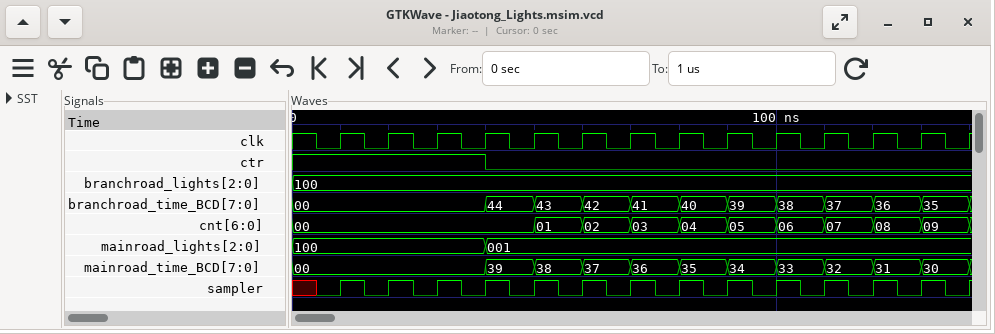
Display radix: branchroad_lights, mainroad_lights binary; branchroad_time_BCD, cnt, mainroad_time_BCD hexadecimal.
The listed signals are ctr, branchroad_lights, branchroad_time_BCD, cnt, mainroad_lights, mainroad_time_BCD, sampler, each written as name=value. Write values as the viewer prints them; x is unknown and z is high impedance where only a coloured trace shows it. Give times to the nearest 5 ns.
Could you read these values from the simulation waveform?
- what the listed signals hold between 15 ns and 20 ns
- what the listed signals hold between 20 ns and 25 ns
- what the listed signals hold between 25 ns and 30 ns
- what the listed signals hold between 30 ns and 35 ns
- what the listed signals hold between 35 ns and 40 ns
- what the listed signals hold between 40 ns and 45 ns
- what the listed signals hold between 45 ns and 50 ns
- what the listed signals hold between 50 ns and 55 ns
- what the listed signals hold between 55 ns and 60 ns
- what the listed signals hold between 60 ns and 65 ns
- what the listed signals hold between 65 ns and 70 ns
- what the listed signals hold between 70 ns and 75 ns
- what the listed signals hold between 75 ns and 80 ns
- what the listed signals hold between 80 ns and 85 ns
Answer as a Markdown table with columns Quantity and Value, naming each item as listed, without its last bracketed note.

| Quantity | Value |
|---|---|
| what the listed signals hold between 15 ns and 20 ns | ctr=1, branchroad_lights=100, branchroad_time_BCD=00, cnt=00, mainroad_lights=100, mainroad_time_BCD=00, sampler=0 |
| what the listed signals hold between 20 ns and 25 ns | ctr=1, branchroad_lights=100, branchroad_time_BCD=00, cnt=00, mainroad_lights=100, mainroad_time_BCD=00, sampler=1 |
| what the listed signals hold between 25 ns and 30 ns | ctr=1, branchroad_lights=100, branchroad_time_BCD=00, cnt=00, mainroad_lights=100, mainroad_time_BCD=00, sampler=0 |
| what the listed signals hold between 30 ns and 35 ns | ctr=1, branchroad_lights=100, branchroad_time_BCD=00, cnt=00, mainroad_lights=100, mainroad_time_BCD=00, sampler=1 |
| what the listed signals hold between 35 ns and 40 ns | ctr=1, branchroad_lights=100, branchroad_time_BCD=00, cnt=00, mainroad_lights=100, mainroad_time_BCD=00, sampler=0 |
| what the listed signals hold between 40 ns and 45 ns | ctr=0, branchroad_lights=100, branchroad_time_BCD=44, cnt=00, mainroad_lights=001, mainroad_time_BCD=39, sampler=1 |
| what the listed signals hold between 45 ns and 50 ns | ctr=0, branchroad_lights=100, branchroad_time_BCD=44, cnt=00, mainroad_lights=001, mainroad_time_BCD=39, sampler=0 |
| what the listed signals hold between 50 ns and 55 ns | ctr=0, branchroad_lights=100, branchroad_time_BCD=43, cnt=01, mainroad_lights=001, mainroad_time_BCD=38, sampler=1 |
| what the listed signals hold between 55 ns and 60 ns | ctr=0, branchroad_lights=100, branchroad_time_BCD=43, cnt=01, mainroad_lights=001, mainroad_time_BCD=38, sampler=0 |
| what the listed signals hold between 60 ns and 65 ns | ctr=0, branchroad_lights=100, branchroad_time_BCD=42, cnt=02, mainroad_lights=001, mainroad_time_BCD=37, sampler=1 |
| what the listed signals hold between 65 ns and 70 ns | ctr=0, branchroad_lights=100, branchroad_time_BCD=42, cnt=02, mainroad_lights=001, mainroad_time_BCD=37, sampler=0 |
| what the listed signals hold between 70 ns and 75 ns | ctr=0, branchroad_lights=100, branchroad_time_BCD=41, cnt=03, mainroad_lights=001, mainroad_time_BCD=36, sampler=1 |
| what the listed signals hold between 75 ns and 80 ns | ctr=0, branchroad_lights=100, branchroad_time_BCD=41, cnt=03, mainroad_lights=001, mainroad_time_BCD=36, sampler=0 |
| what the listed signals hold between 80 ns and 85 ns | ctr=0, branchroad_lights=100, branchroad_time_BCD=40, cnt=04, mainroad_lights=001, mainroad_time_BCD=35, sampler=1 |
